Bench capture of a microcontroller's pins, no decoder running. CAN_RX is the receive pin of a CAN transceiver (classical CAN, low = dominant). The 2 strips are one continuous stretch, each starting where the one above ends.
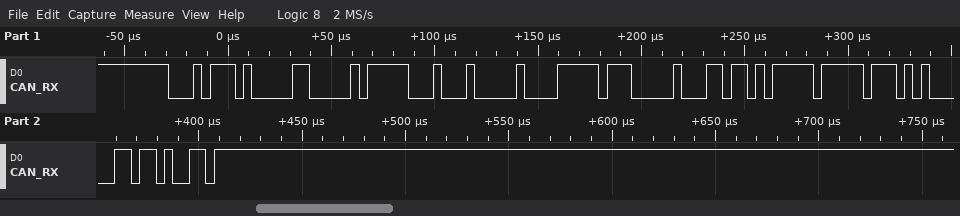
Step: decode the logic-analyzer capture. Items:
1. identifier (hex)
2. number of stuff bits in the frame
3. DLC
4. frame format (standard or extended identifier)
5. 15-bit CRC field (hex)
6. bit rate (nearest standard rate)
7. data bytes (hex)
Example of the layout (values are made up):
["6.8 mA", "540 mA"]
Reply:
["0x174", "9", "8", "standard", "0x4169", "250 kbit/s", "1F 22 00 FF 00 DA FF FA"]
